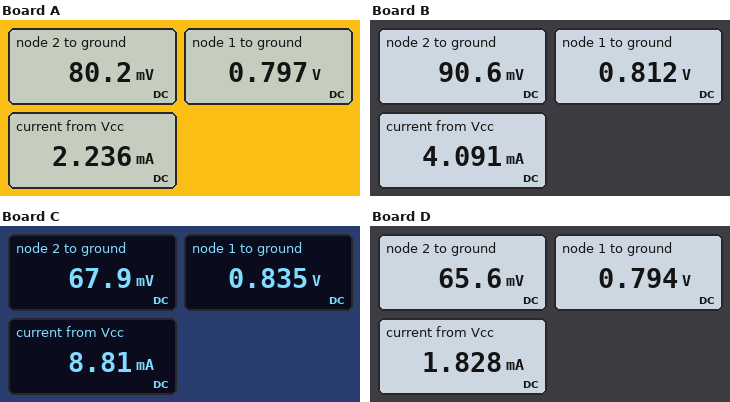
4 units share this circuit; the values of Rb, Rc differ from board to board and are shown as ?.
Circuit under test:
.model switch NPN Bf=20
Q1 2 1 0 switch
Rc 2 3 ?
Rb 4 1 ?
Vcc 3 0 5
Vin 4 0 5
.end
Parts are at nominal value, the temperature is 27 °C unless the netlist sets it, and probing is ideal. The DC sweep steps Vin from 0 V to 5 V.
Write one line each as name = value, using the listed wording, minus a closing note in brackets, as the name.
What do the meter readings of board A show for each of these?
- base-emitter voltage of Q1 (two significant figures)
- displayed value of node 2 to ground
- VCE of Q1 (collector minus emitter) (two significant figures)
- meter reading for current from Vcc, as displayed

base-emitter voltage of Q1 = 800 mV
displayed value of node 2 to ground = 80.2 mV
VCE of Q1 (collector minus emitter) = 80 mV
meter reading for current from Vcc, as displayed = 2.236 mA
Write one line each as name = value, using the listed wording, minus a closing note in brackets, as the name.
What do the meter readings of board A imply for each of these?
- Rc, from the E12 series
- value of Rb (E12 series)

Rc, from the E12 series = 2.2 kΩ
value of Rb = 18 kΩ
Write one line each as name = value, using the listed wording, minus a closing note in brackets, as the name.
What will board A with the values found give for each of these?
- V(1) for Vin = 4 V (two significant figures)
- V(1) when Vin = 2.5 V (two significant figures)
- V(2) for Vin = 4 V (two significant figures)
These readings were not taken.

V(1) for Vin = 4 V = 800 mV
V(1) when Vin = 2.5 V = 790 mV
V(2) for Vin = 4 V = 95 mV
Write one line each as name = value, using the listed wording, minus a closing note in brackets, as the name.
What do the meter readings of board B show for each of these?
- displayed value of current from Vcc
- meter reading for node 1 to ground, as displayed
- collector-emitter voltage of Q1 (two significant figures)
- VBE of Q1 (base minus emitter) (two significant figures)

displayed value of current from Vcc = 4.091 mA
meter reading for node 1 to ground, as displayed = 0.812 V
collector-emitter voltage of Q1 = 91 mV
VBE of Q1 (base minus emitter) = 810 mV
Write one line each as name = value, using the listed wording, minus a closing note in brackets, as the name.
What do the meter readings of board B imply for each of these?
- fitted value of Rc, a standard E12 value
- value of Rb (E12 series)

fitted value of Rc, a standard E12 value = 1.2 kΩ
value of Rb = 12 kΩ
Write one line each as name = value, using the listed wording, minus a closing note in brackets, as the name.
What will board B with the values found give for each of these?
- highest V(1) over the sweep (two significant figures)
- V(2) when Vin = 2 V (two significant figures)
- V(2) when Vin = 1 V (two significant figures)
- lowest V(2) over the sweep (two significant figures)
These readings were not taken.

highest V(1) over the sweep = 810 mV
V(2) when Vin = 2 V = 2.6 V
V(2) when Vin = 1 V = 4.5 V
lowest V(2) over the sweep = 91 mV
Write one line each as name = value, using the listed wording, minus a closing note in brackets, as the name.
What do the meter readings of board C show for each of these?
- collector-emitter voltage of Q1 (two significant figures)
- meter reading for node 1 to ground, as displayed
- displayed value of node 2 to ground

collector-emitter voltage of Q1 = 68 mV
meter reading for node 1 to ground, as displayed = 0.835 V
displayed value of node 2 to ground = 67.9 mV
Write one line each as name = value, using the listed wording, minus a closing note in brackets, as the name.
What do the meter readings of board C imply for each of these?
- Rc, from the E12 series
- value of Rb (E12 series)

Rc, from the E12 series = 560 Ω
value of Rb = 3.3 kΩ
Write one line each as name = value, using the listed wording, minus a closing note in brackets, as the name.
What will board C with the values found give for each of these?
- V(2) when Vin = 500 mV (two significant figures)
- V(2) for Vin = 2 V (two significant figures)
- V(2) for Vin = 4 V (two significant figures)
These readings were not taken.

V(2) when Vin = 500 mV = 5.0 V
V(2) for Vin = 2 V = 1.0 V
V(2) for Vin = 4 V = 78 mV
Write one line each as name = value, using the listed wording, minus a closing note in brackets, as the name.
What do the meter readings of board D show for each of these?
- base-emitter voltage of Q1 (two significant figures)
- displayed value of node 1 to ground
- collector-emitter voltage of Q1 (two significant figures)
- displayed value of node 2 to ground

base-emitter voltage of Q1 = 790 mV
displayed value of node 1 to ground = 0.794 V
collector-emitter voltage of Q1 = 66 mV
displayed value of node 2 to ground = 65.6 mV
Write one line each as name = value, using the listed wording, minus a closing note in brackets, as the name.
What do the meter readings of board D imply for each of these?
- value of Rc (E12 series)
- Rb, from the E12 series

value of Rc = 2.7 kΩ
Rb, from the E12 series = 15 kΩ
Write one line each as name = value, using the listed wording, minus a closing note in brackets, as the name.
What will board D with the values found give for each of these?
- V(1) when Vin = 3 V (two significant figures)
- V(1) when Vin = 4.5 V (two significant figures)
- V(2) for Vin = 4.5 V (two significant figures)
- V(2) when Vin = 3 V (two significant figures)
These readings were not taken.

V(1) when Vin = 3 V = 790 mV
V(1) when Vin = 4.5 V = 790 mV
V(2) for Vin = 4.5 V = 70 mV
V(2) when Vin = 3 V = 94 mV
